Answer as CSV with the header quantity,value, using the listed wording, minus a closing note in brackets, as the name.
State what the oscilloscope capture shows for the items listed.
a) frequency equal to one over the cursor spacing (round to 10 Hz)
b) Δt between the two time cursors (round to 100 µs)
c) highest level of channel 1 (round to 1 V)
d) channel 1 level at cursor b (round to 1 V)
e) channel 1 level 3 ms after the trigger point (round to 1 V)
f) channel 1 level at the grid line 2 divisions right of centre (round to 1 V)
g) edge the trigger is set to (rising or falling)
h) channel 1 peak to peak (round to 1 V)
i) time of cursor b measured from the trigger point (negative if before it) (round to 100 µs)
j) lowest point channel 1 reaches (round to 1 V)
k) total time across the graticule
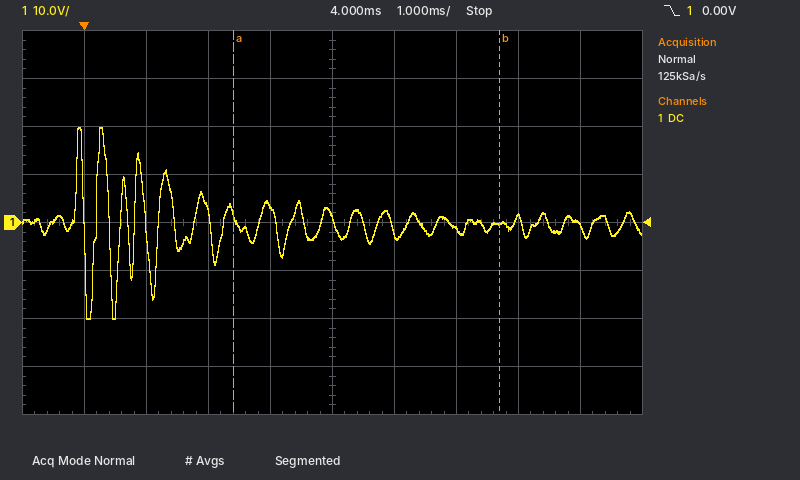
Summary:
quantity,value
frequency equal to one over the cursor spacing,230 Hz
Δt between the two time cursors,4.3 ms
highest level of channel 1,20 V
channel 1 level at cursor b,0 V
channel 1 level 3 ms after the trigger point,4 V
channel 1 level at the grid line 2 divisions right of centre,-1 V
edge the trigger is set to,falling
channel 1 peak to peak,40 V
time of cursor b measured from the trigger point (negative if before it),+6.7 ms
lowest point channel 1 reaches,-20 V
total time across the graticule,10 ms
